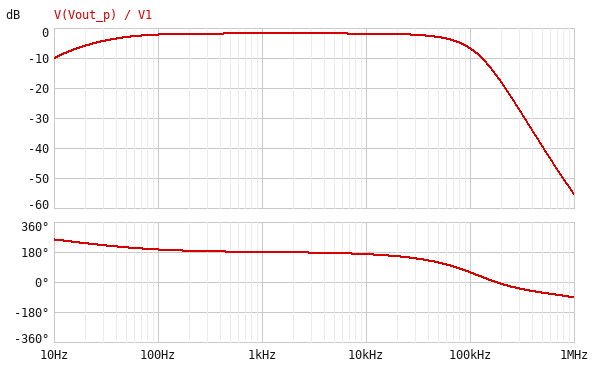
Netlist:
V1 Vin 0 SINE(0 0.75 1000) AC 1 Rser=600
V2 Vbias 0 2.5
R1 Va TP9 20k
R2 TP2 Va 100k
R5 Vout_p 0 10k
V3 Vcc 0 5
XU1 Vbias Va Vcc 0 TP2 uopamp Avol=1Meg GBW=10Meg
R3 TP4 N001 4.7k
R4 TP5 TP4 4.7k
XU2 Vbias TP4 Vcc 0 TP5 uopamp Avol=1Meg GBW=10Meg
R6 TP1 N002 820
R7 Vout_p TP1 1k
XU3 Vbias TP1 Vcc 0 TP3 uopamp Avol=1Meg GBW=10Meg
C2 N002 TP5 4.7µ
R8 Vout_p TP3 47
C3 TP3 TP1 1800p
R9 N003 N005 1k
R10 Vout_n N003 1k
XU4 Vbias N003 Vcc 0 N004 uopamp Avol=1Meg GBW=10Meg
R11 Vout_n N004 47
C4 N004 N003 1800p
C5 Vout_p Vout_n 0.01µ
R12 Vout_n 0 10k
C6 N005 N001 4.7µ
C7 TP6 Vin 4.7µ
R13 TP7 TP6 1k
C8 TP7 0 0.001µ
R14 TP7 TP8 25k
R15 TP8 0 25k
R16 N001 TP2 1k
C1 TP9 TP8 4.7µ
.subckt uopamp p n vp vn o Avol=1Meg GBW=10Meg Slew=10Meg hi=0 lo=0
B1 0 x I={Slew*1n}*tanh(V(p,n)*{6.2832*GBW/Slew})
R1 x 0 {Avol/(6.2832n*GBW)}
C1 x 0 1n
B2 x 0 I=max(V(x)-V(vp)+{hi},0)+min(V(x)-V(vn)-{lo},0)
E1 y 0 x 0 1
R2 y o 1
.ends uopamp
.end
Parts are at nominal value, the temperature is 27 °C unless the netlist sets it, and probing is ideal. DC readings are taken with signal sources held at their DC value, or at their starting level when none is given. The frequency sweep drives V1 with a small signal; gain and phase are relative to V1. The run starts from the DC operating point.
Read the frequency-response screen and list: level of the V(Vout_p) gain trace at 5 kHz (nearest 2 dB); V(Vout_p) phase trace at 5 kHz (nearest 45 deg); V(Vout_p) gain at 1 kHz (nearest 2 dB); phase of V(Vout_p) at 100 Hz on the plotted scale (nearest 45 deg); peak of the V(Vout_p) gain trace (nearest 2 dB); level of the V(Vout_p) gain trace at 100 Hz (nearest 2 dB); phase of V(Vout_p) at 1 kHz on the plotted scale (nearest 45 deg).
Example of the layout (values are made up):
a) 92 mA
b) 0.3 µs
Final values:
a) -2 dB
b) 180 deg
c) -2 dB
d) 180 deg
e) -2 dB
f) -2 dB
g) 180 deg
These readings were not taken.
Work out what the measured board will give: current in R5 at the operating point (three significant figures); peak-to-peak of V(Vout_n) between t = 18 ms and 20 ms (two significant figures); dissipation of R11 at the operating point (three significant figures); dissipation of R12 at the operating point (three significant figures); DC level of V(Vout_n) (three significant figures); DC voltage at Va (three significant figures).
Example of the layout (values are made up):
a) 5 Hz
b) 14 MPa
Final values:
a) 250 µA
b) 1.0 V
c) 2.94 µW
d) 625 µW
e) 2.50 V
f) 2.50 V
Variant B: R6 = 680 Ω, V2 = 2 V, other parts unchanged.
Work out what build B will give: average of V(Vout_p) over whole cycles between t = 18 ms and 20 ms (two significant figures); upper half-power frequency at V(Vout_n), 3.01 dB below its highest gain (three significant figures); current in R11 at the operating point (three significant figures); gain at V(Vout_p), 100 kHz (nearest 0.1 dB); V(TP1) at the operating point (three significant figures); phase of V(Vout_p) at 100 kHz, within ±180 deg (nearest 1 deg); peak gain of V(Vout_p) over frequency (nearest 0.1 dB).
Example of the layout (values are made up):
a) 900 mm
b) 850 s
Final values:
a) 2.0 V
b) 86.6 kHz
c) 200 µA
d) -5.3 dB
e) 2.00 V
f) 60 deg
g) -0.2 dB
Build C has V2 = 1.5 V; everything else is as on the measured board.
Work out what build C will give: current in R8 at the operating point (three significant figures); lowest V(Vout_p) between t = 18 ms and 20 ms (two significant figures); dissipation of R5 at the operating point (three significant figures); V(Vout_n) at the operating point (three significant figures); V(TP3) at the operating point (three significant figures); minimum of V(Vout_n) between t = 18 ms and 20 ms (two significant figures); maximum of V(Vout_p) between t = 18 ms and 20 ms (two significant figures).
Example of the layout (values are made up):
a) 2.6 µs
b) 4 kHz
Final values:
a) 150 µA
b) 890 mV
c) 225 µW
d) 1.50 V
e) 1.51 V
f) 1.0 V
g) 2.1 V
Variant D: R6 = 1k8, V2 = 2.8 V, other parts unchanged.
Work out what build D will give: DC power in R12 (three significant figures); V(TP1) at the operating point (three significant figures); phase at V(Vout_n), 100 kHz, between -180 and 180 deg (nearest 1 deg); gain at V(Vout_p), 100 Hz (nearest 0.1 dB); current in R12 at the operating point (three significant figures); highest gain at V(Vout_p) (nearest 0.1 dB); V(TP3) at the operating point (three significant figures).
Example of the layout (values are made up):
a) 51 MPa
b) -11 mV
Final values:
a) 784 µW
b) 2.80 V
c) -117 deg
d) -8.5 dB
e) 280 µA
f) -7.9 dB
g) 2.81 V
